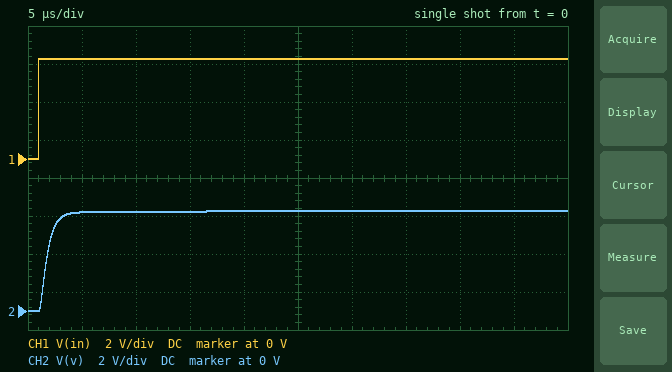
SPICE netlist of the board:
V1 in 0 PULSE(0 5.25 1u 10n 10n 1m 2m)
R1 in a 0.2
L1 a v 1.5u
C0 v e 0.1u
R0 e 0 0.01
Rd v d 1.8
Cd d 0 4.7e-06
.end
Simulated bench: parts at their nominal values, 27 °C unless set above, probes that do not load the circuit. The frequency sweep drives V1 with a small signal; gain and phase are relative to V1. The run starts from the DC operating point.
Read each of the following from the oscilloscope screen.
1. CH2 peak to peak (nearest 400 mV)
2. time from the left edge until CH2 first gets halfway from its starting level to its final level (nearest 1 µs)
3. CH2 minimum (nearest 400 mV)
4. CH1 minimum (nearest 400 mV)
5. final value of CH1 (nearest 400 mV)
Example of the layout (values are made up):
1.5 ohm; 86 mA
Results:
5.2 V; 2 µs; 0 V; 0 V; 5.2 V
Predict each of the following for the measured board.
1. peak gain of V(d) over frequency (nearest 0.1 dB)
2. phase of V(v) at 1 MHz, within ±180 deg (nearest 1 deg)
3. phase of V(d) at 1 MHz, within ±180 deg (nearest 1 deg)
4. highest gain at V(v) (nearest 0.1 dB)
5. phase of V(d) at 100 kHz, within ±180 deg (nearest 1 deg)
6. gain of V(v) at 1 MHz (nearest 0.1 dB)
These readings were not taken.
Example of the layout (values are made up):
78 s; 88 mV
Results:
0 dB; -132 deg; 139 deg; 0 dB; -109 deg; -17.3 dB
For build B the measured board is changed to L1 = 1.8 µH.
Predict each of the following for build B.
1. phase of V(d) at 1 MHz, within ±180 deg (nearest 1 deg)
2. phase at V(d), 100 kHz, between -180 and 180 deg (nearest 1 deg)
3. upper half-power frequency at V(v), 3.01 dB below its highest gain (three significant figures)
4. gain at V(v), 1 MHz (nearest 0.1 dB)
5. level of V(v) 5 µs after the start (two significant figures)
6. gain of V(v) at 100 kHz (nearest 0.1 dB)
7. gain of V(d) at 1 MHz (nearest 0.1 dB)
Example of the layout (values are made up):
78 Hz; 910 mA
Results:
138 deg; -114 deg; 188 kHz; -19.0 dB; 5.2 V; -1.0 dB; -53.5 dB
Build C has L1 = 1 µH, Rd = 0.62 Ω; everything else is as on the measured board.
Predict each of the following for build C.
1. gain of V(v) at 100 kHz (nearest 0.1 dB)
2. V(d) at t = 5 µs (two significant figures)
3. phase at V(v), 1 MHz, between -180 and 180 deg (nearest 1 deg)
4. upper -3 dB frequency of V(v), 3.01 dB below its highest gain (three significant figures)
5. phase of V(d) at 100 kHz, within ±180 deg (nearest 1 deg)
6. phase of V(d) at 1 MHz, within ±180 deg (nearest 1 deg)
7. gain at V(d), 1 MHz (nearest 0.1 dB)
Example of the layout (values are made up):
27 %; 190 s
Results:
-1.7 dB; 3.1 V; -107 deg; 119 kHz; -111 deg; 166 deg; -45.9 dB
